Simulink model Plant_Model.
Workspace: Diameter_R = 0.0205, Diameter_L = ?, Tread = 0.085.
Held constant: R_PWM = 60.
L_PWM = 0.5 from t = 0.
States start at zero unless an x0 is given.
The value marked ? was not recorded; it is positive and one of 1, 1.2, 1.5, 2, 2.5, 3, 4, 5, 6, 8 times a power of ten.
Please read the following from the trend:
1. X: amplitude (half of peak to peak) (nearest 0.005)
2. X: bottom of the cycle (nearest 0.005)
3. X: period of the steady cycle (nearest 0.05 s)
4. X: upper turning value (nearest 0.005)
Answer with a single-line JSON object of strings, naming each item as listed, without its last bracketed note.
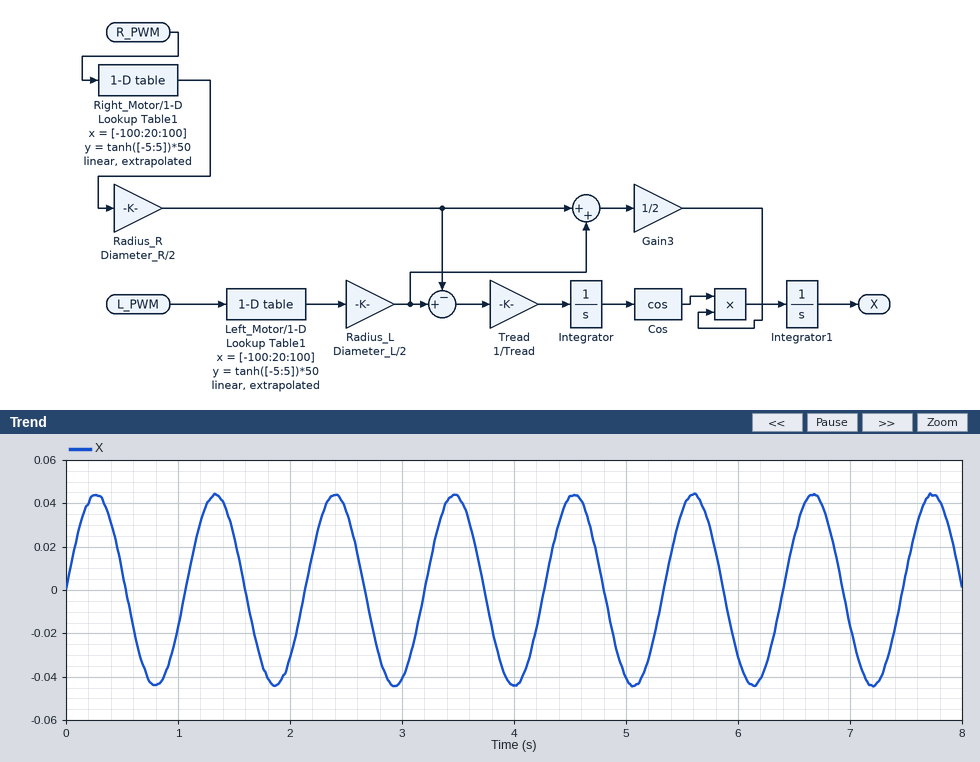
{"X: amplitude (half of peak to peak)": "0.045", "X: bottom of the cycle": "-0.045", "X: period of the steady cycle": "1.05 s", "X: upper turning value": "0.045"}
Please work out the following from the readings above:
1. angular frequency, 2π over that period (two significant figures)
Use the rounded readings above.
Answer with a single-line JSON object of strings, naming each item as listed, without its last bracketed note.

{"angular frequency, 2π over that period": "6.0 rad/s"}
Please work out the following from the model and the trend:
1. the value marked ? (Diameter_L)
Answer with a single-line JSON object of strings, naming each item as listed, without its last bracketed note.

{"the value marked ?": "0.02"}
